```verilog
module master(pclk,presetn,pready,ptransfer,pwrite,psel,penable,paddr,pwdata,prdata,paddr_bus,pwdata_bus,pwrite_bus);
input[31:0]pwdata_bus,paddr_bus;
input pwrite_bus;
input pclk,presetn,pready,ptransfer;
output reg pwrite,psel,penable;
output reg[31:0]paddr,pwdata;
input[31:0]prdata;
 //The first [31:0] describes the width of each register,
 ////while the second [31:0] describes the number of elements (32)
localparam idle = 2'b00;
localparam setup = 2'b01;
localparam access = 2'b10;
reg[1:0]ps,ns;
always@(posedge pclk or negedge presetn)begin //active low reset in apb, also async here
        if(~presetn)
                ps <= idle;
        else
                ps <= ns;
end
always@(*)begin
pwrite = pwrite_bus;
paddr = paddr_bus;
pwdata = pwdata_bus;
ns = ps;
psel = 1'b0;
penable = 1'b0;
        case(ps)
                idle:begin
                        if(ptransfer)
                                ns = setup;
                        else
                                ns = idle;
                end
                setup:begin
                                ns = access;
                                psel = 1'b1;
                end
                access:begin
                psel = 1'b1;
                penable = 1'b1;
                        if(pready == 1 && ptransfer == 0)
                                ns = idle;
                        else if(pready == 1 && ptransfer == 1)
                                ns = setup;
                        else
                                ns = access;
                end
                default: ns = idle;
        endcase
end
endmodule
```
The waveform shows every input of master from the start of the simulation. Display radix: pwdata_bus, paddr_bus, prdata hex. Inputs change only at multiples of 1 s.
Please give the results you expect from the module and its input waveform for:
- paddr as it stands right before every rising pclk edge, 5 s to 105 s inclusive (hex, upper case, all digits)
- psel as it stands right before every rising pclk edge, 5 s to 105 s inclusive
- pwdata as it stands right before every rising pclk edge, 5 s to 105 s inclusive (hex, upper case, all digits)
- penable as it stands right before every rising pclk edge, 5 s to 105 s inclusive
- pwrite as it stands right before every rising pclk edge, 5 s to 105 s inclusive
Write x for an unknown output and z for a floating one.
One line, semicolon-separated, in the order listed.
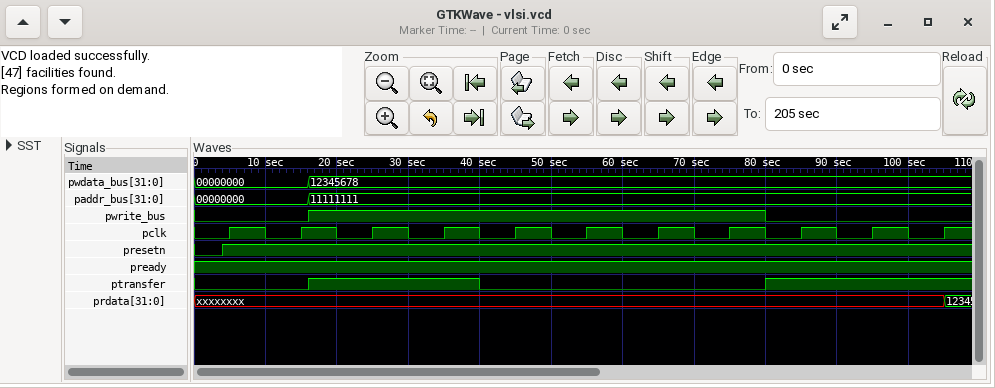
00000000, 00000000, 11111111, 11111111, 11111111, 11111111, 11111111, 11111111, 11111111, 11111111, 11111111; 0 0 0 1 1 0 0 0 0 1 1; 00000000, 00000000, 12345678, 12345678, 12345678, 12345678, 12345678, 12345678, 12345678, 12345678, 12345678; 0 0 0 0 1 0 0 0 0 0 1; 0 0 1 1 1 1 1 1 0 0 0
